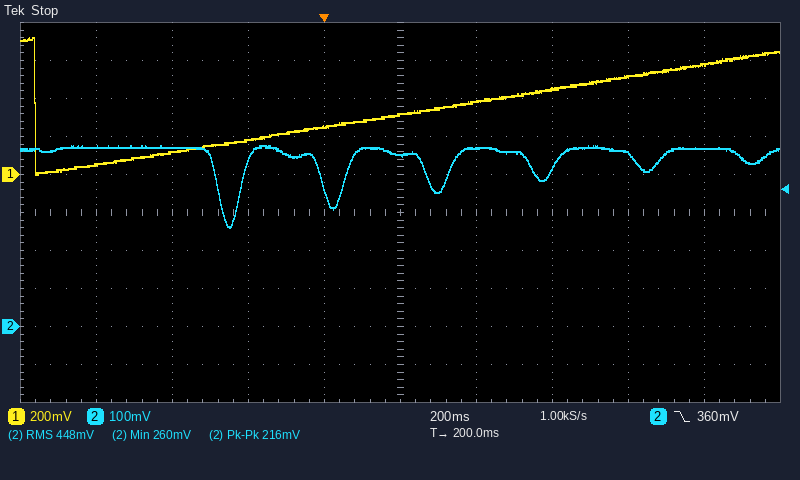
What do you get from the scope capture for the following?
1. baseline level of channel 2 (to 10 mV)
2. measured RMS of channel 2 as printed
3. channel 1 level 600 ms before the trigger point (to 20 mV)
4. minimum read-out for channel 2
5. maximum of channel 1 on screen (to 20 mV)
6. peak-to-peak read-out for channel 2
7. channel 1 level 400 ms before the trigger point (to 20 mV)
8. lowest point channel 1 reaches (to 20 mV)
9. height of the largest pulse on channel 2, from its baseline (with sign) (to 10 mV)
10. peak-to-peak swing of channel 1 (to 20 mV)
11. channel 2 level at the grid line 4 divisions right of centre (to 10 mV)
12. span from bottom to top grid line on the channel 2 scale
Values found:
470 mV
448 mV
60 mV
260 mV
720 mV
216 mV
120 mV
0 mV
-210 mV
720 mV
470 mV
1 V
